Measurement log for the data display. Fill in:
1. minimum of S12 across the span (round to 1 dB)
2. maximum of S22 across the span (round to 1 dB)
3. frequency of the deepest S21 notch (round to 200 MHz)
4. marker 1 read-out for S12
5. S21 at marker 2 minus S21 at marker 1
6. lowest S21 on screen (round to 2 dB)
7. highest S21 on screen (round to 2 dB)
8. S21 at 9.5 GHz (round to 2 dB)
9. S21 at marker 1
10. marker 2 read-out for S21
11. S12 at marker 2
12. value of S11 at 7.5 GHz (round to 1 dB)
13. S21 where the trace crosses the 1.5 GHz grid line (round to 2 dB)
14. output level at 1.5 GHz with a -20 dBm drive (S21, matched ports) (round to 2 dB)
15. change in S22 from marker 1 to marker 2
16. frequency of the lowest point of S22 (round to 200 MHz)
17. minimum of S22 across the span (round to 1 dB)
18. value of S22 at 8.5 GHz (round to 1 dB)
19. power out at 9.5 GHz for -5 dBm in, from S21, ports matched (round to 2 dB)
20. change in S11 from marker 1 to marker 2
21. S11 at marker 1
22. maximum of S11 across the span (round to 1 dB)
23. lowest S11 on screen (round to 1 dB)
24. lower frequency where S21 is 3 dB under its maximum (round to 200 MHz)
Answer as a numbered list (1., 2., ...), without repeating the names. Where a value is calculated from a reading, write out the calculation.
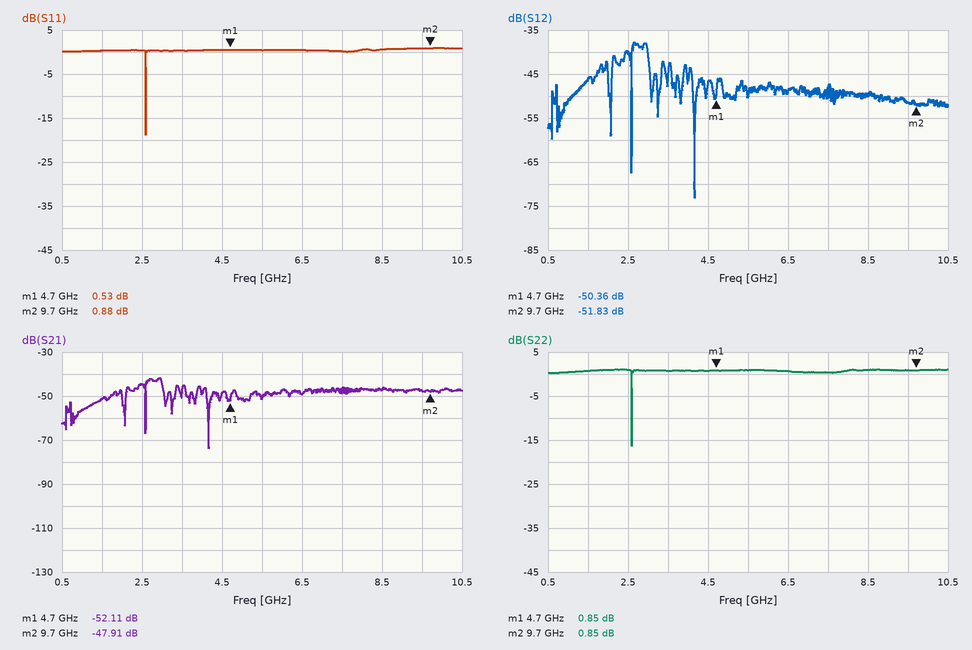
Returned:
1. -73 dB
2. 1 dB
3. 4.2 GHz
4. -50.36 dB
5. -47.91 − (-52.11) = 4.20 dB
6. -74 dB
7. -42 dB
8. -48 dB
9. -52.11 dB
10. -47.91 dB
11. -51.83 dB
12. 0 dB
13. -52 dB
14. -20 dBm + (-52 dB) = -72 dBm
15. 0.85 − (0.85) = 0.00 dB
16. 2.6 GHz
17. -16 dB
18. 1 dB
19. -5 dBm + (-48 dB) = -52 dBm
20. 0.88 − (0.53) = 0.35 dB
21. 0.53 dB
22. 1 dB
23. -19 dB
24. 2.6 GHz
